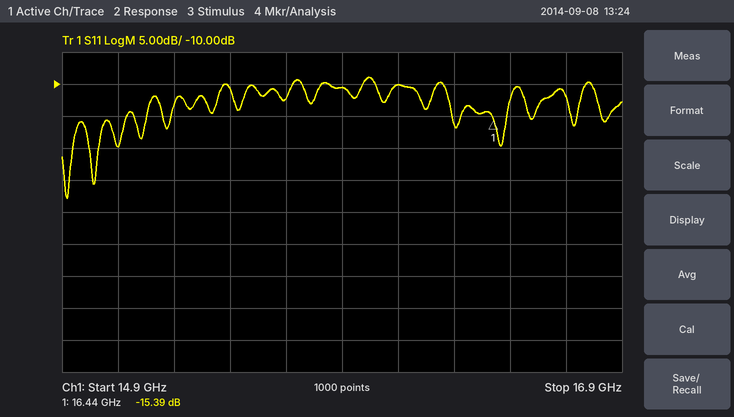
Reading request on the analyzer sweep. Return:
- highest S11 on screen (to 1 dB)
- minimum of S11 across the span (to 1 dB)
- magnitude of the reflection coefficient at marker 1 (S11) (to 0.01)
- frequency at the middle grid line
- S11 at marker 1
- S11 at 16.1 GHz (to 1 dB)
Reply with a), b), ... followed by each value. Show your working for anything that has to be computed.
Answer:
a) -9 dB
b) -28 dB
c) 10^(-15.39/20) ≈ 0.17
d) 15.9 GHz
e) -15.39 dB
f) -10 dB
